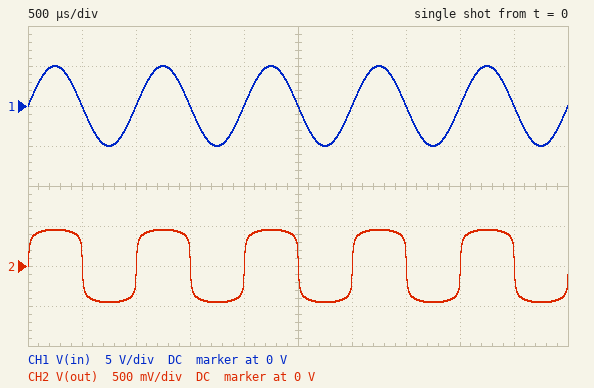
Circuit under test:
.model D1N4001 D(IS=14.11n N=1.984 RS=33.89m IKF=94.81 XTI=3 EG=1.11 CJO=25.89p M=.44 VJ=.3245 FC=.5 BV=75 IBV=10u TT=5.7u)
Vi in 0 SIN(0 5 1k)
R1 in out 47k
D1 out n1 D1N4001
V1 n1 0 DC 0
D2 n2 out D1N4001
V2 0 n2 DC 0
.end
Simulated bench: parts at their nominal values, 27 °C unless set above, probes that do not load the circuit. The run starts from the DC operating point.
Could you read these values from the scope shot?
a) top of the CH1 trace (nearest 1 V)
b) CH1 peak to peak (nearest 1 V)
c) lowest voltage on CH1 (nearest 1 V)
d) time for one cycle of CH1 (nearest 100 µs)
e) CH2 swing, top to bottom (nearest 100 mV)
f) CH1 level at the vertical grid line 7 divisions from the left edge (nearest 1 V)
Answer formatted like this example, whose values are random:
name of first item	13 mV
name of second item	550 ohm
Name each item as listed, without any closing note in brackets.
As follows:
top of the CH1 trace	5 V
CH1 peak to peak	10 V
lowest voltage on CH1	-5 V
time for one cycle of CH1	1.0 ms
CH2 swing, top to bottom	900 mV
CH1 level at the vertical grid line 7 divisions from the left edge	0 V
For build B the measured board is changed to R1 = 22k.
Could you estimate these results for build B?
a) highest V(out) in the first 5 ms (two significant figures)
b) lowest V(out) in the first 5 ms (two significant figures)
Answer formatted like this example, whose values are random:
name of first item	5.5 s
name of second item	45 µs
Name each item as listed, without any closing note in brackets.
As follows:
highest V(out) in the first 5 ms	490 mV
lowest V(out) in the first 5 ms	-490 mV
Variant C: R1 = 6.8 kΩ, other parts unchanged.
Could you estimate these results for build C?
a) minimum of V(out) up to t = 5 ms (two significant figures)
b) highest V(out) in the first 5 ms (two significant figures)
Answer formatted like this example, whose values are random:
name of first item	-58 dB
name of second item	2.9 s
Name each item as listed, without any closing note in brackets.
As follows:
minimum of V(out) up to t = 5 ms	-550 mV
highest V(out) in the first 5 ms	550 mV
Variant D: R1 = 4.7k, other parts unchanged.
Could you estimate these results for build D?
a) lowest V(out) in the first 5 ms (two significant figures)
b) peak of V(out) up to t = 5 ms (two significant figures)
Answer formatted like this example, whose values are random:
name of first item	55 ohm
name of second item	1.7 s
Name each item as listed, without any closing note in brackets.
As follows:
lowest V(out) in the first 5 ms	-570 mV
peak of V(out) up to t = 5 ms	570 mV
